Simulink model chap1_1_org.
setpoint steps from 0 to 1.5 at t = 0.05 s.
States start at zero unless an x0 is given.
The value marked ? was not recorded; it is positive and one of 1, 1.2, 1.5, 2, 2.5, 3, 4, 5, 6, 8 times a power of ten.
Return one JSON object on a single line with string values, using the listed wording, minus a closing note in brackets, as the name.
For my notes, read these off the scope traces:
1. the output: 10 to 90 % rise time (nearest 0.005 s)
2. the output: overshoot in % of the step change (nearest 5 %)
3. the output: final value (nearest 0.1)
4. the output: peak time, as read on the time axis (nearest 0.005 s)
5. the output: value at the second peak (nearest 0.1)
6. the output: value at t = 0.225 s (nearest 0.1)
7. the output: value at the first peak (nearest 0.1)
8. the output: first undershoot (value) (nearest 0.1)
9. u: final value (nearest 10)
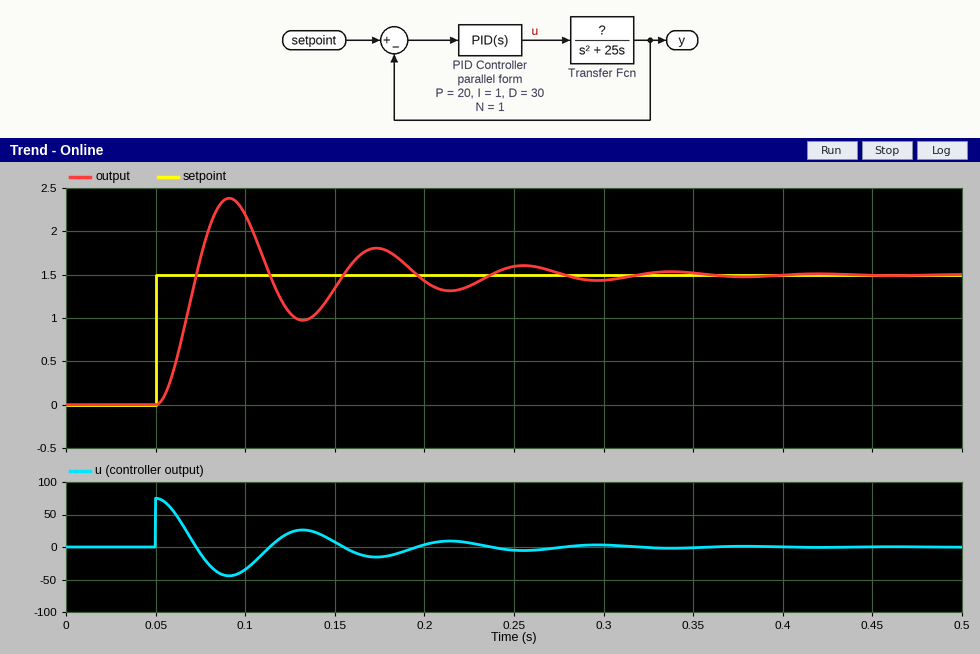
{"the output: 10 to 90 % rise time": "0.015 s", "the output: overshoot in % of the step change": "60 %", "the output: final value": "1.5", "the output: peak time, as read on the time axis": "0.090 s", "the output: value at the second peak": "1.8", "the output: value at t = 0.225 s": "1.4", "the output: value at the first peak": "2.4", "the output: first undershoot (value)": "1.0", "u: final value": "0"}
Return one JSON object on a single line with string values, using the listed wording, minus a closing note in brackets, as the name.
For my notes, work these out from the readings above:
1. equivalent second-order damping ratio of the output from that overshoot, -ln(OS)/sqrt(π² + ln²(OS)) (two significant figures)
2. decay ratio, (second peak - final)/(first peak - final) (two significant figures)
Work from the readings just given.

{"equivalent second-order damping ratio of the output from that overshoot, -ln(OS)/sqrt(π² + ln²(OS))": "0.16", "decay ratio, (second peak - final)/(first peak - final)": "0.33"}
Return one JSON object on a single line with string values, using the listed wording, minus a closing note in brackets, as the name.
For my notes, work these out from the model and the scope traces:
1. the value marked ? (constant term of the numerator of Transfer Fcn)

{"the value marked ?": "120"}
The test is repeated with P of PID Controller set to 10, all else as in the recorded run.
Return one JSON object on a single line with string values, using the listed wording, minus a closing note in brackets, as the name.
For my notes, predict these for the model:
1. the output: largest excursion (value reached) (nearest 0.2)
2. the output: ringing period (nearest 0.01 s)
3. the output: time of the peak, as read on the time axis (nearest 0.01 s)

{"the output: largest excursion (value reached)": "2.4", "the output: ringing period": "0.09 s", "the output: time of the peak, as read on the time axis": "0.10 s"}
